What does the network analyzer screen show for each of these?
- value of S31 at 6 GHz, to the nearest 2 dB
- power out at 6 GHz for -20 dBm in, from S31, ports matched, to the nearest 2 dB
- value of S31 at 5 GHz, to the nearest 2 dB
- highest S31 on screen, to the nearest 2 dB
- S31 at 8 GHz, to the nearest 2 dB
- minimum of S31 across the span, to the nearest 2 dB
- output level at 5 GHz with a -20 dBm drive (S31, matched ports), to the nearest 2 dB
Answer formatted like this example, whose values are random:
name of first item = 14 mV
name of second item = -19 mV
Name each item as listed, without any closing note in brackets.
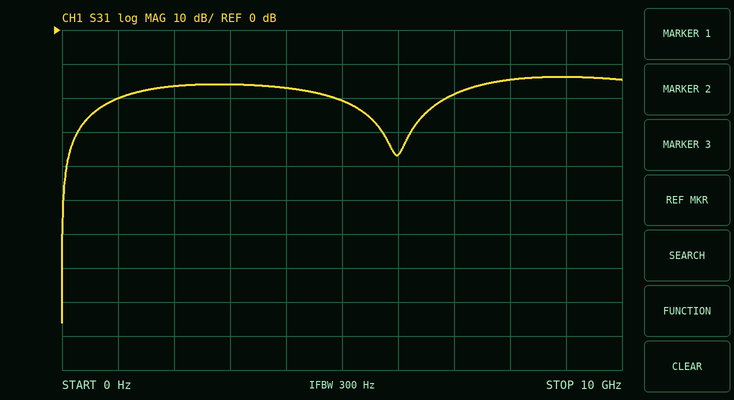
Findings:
value of S31 at 6 GHz, to the nearest 2 dB = -36 dB
power out at 6 GHz for -20 dBm in, from S31, ports matched, to the nearest 2 dB = -56 dBm
value of S31 at 5 GHz, to the nearest 2 dB = -20 dB
highest S31 on screen, to the nearest 2 dB = -14 dB
S31 at 8 GHz, to the nearest 2 dB = -14 dB
minimum of S31 across the span, to the nearest 2 dB = -86 dB
output level at 5 GHz with a -20 dBm drive (S31, matched ports), to the nearest 2 dB = -40 dBm
